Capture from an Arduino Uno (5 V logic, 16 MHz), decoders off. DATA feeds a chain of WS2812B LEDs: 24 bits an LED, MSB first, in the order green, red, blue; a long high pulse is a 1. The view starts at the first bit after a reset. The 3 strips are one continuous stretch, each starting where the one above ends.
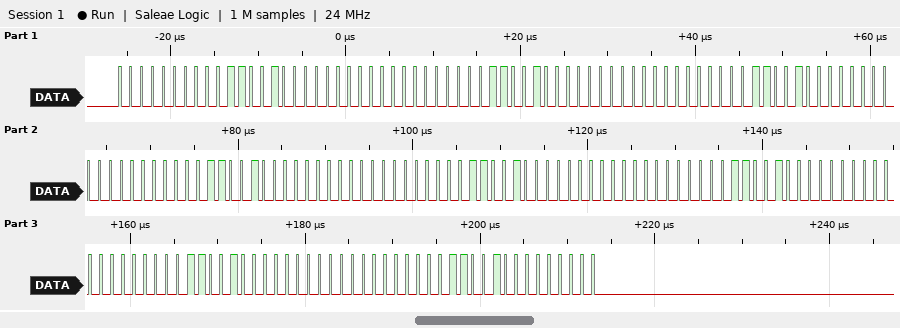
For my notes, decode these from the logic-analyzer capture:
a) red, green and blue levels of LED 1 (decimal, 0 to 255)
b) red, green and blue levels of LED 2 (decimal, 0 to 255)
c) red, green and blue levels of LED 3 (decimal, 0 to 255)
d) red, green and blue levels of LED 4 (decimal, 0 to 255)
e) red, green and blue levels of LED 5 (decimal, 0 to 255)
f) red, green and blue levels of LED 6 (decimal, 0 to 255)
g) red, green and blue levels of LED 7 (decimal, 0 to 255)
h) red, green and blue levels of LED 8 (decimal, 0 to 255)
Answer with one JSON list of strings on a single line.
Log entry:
["50, 0, 0", "50, 0, 0", "50, 0, 0", "50, 0, 0", "50, 0, 0", "50, 0, 0", "50, 0, 0", "50, 0, 0"]
